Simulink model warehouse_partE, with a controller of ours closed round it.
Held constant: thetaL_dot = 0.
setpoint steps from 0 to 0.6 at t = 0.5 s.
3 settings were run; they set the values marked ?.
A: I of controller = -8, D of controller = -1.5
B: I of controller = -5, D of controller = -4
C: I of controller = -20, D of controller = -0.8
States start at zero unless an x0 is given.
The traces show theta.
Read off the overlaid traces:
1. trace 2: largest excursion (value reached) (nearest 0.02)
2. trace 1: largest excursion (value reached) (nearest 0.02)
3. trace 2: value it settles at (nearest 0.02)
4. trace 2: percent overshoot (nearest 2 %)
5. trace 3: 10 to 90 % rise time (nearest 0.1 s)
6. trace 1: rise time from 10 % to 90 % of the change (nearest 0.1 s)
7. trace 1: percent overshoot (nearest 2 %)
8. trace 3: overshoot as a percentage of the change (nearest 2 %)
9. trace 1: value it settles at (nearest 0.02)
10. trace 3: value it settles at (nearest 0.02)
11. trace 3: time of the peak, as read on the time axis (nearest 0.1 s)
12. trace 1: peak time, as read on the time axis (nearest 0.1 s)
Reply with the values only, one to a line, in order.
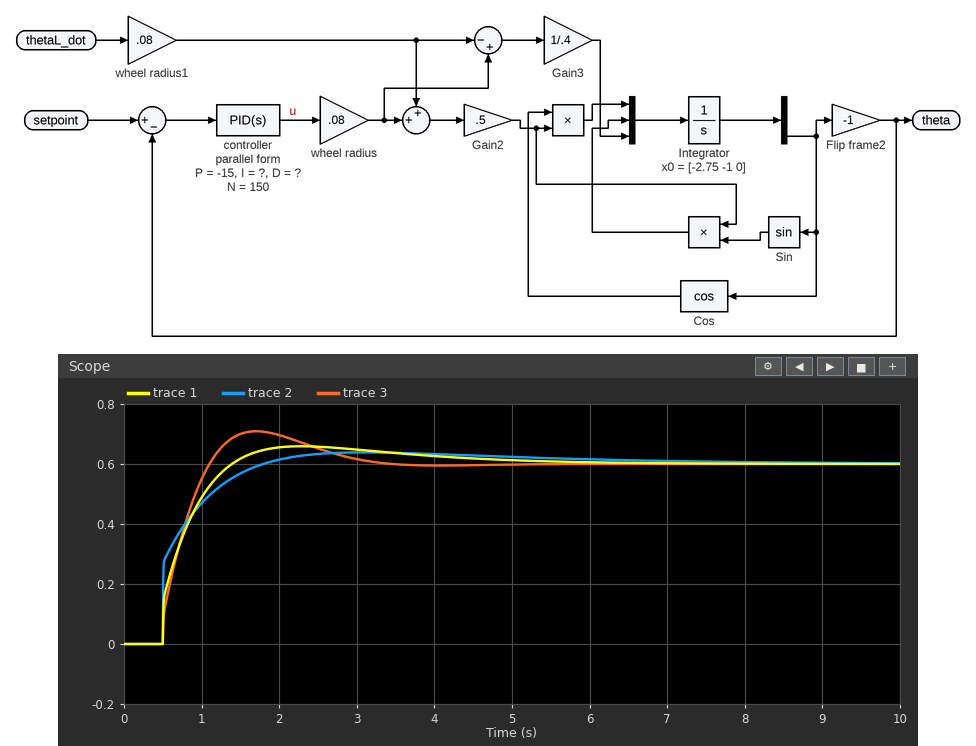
0.64
0.66
0.60
6 %
0.5 s
0.6 s
10 %
18 %
0.60
0.60
1.7 s
2.3 s
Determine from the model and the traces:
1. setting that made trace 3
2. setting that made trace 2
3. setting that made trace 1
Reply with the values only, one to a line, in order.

C
B
A
